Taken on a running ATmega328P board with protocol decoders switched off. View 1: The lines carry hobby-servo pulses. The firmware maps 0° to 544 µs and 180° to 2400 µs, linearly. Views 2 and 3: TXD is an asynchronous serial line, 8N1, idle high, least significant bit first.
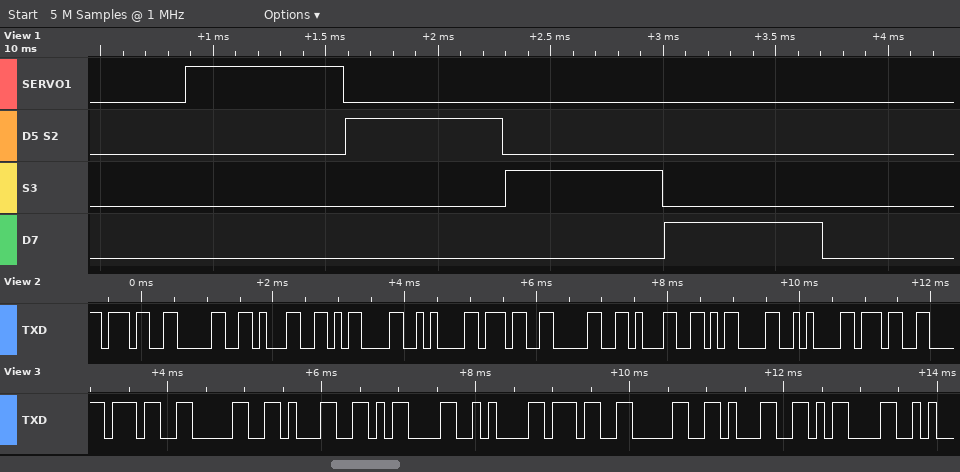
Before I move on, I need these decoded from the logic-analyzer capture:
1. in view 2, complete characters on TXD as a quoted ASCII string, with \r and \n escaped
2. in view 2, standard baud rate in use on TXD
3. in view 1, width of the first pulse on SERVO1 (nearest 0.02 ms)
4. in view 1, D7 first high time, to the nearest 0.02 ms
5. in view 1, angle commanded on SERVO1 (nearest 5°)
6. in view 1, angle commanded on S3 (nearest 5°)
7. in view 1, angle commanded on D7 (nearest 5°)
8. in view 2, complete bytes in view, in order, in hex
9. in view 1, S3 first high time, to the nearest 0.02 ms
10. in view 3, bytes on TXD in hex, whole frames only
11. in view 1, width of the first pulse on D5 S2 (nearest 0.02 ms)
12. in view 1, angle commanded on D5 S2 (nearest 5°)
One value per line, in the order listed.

"701\r\n701\r\n7"
9600 baud
0.70 ms
0.70 ms
15°
15°
15°
37 30 31 0D 0A 37 30 31 0D 0A 37
0.70 ms
0x37 0x30 0x31 0x0D 0x0A 0x37 0x30 0x31 0x0D
0.70 ms
15°
